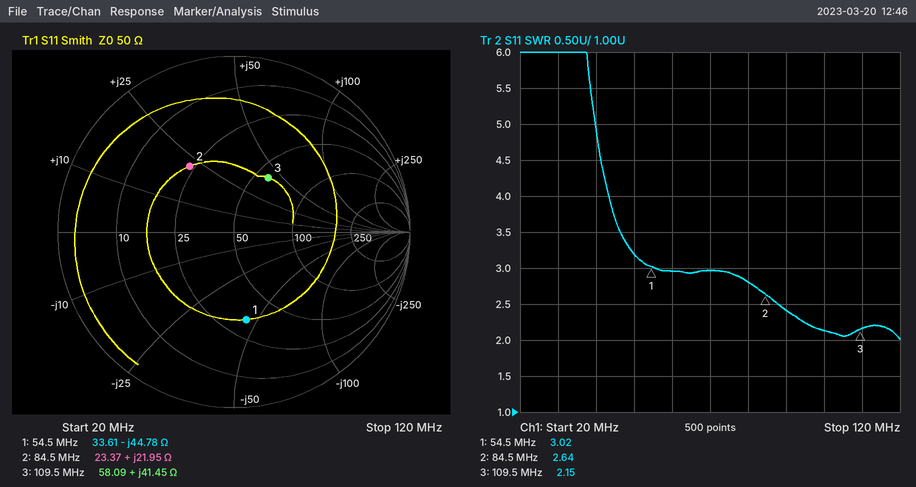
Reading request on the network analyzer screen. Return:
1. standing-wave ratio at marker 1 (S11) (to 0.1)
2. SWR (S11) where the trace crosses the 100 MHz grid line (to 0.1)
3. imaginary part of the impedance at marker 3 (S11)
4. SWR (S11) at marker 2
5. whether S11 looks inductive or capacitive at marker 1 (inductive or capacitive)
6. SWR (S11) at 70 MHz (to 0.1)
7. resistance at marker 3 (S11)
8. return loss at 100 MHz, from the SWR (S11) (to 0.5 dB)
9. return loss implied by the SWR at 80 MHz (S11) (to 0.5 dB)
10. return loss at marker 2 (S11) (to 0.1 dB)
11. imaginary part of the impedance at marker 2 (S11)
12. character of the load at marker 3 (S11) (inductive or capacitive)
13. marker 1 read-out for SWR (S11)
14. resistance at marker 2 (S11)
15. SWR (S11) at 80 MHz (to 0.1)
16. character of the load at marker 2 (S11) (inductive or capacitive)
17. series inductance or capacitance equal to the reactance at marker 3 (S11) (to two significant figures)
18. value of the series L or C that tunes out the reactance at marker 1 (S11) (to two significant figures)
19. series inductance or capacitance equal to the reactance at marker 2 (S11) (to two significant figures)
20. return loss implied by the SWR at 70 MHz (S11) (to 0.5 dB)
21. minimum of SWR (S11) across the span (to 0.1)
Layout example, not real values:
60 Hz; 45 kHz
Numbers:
3.0; 2.1; +41.45 Ω; 2.64; capacitive; 3.0; 58.09 Ω; 9.0 dB; 6.5 dB; 6.9 dB; +21.95 Ω; inductive; 3.02; 23.37 Ω; 2.8; inductive; 60 nH; 130 nH; 41 nH; 6.0 dB; 2.0
